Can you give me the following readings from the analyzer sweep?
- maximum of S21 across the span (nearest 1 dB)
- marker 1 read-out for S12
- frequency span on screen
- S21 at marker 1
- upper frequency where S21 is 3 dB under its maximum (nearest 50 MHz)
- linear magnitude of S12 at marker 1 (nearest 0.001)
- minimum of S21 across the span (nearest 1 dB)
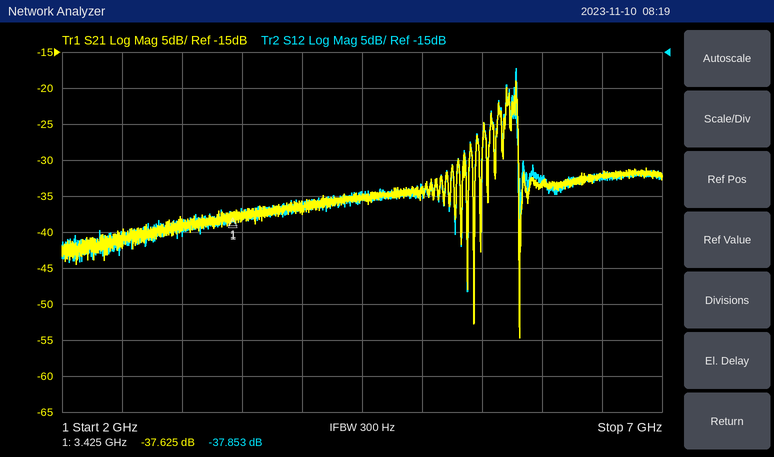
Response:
-19 dB
-37.853 dB
5 GHz
-37.625 dB
5.80 GHz
0.013
-55 dB
